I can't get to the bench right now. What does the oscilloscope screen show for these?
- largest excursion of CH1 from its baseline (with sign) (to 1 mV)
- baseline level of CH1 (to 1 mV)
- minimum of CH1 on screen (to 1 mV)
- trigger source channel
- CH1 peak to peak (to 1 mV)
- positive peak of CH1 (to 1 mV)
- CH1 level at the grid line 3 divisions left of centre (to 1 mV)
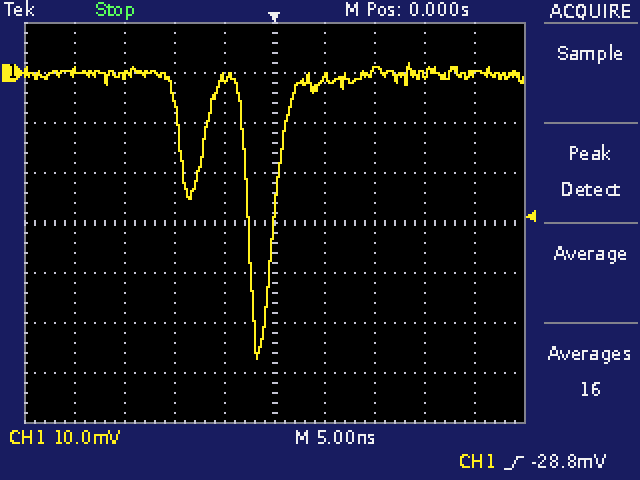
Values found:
-57 mV
0 mV
-57 mV
CH1
59 mV
2 mV
0 mV
